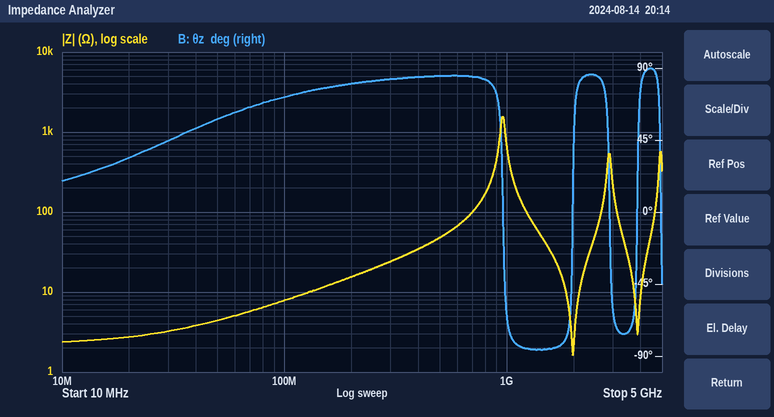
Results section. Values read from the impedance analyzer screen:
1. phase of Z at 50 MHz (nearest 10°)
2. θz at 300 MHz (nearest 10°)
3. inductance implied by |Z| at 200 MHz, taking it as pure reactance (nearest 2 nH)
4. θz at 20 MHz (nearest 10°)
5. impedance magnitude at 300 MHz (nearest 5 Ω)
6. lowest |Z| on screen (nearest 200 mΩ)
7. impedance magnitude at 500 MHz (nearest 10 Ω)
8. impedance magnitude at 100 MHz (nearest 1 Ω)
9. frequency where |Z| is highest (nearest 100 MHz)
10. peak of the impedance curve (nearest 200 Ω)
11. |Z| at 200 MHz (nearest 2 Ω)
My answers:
60°
80°
12 nH
30°
25 Ω
1.6 Ω
50 Ω
8 Ω
1.0 GHz
1.6 kΩ
16 Ω
